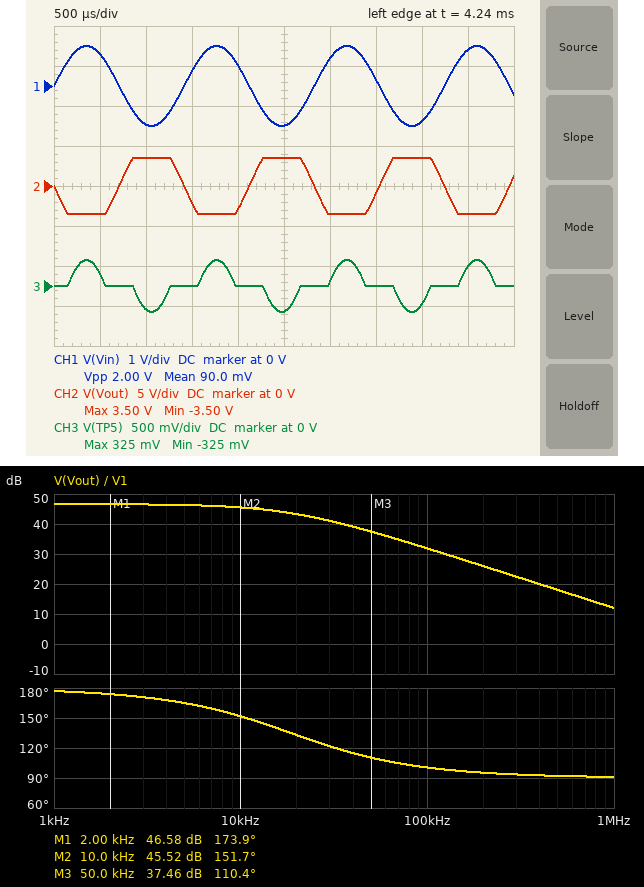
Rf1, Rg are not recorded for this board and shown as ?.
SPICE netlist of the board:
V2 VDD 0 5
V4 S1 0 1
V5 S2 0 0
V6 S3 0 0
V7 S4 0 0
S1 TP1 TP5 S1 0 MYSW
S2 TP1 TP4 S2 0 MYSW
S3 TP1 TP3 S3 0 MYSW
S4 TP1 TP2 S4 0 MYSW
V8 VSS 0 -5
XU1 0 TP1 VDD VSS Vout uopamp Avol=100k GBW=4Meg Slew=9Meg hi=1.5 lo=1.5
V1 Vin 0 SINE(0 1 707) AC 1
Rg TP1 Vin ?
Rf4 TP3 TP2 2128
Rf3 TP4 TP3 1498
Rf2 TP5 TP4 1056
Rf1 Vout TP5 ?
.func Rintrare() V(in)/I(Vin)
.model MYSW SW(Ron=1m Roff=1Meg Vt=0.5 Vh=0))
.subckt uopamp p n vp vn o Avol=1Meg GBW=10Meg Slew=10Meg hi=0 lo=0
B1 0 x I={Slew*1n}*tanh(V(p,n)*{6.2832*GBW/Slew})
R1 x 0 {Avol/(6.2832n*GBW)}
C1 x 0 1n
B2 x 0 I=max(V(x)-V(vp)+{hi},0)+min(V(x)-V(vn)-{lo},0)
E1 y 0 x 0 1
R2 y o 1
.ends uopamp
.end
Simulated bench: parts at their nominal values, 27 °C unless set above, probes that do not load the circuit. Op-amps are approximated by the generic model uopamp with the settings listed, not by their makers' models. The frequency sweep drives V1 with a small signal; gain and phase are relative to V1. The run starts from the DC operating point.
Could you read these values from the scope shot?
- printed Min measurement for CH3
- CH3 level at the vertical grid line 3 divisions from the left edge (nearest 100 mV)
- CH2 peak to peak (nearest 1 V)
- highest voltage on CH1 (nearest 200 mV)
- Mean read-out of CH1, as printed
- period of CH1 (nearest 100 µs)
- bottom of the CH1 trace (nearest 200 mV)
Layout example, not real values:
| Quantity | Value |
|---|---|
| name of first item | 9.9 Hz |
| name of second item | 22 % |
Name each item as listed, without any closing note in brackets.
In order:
| Quantity | Value |
|---|---|
| printed Min measurement for CH3 | -325 mV |
| CH3 level at the vertical grid line 3 divisions from the left edge | 0 V |
| CH2 peak to peak | 7 V |
| highest voltage on CH1 | 1.0 V |
| Mean read-out of CH1, as printed | 90.0 mV |
| period of CH1 | 1.4 ms |
| bottom of the CH1 trace | -1.0 V |
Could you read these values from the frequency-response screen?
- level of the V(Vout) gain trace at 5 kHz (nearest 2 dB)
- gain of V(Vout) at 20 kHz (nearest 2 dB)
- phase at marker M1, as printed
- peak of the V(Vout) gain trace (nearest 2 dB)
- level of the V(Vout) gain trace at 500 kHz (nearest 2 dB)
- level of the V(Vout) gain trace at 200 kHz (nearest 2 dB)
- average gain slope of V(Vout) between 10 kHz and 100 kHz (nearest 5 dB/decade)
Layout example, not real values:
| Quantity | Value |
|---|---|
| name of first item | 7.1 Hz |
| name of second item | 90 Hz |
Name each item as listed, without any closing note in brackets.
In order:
| Quantity | Value |
|---|---|
| level of the V(Vout) gain trace at 5 kHz | 46 dB |
| gain of V(Vout) at 20 kHz | 44 dB |
| phase at marker M1, as printed | 173.9 deg |
| peak of the V(Vout) gain trace | 46 dB |
| level of the V(Vout) gain trace at 500 kHz | 18 dB |
| level of the V(Vout) gain trace at 200 kHz | 26 dB |
| average gain slope of V(Vout) between 10 kHz and 100 kHz | -15 dB/decade |
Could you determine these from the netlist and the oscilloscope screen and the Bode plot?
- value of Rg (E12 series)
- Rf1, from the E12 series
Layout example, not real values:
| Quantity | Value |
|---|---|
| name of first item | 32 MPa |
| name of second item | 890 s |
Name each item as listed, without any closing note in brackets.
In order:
| Quantity | Value |
|---|---|
| value of Rg | 1.2 kΩ |
| Rf1, from the E12 series | 6.8 kΩ |
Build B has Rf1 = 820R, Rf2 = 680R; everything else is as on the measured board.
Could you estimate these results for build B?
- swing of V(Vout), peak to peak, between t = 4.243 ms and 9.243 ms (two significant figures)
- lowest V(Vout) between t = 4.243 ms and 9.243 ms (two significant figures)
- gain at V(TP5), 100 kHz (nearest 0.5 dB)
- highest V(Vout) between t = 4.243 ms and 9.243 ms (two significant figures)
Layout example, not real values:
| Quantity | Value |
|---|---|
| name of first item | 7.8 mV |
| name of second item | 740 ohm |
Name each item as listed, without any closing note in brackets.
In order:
| Quantity | Value |
|---|---|
| swing of V(Vout), peak to peak, between t = 4.243 ms and 9.243 ms | 1.4 V |
| lowest V(Vout) between t = 4.243 ms and 9.243 ms | -680 mV |
| gain at V(TP5), 100 kHz | 32.0 dB |
| highest V(Vout) between t = 4.243 ms and 9.243 ms | 680 mV |
